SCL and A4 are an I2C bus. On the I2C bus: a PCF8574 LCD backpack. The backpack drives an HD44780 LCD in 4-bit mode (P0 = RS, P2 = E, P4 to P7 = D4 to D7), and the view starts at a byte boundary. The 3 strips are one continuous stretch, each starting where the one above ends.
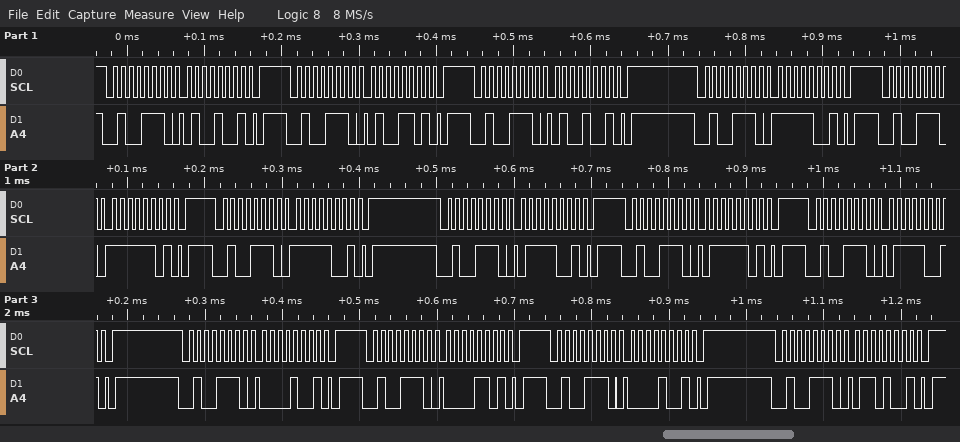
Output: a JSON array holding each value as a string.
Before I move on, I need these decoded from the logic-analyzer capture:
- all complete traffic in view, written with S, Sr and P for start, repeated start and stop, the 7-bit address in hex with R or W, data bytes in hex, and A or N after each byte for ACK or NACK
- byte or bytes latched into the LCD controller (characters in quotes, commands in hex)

["S 27W A 49 A P S 27W A 4D A P S 27W A 49 A P S 27W A F9 A P S 27W A FD A P S 27W A F9 A P S 27W A 79 A P S 27W A 7D A P S 27W A 79 A P S 27W A 09 A P S 27W A 0D A P S 27W A 09 A P S 27W A 69 A P", "'O' 'p'"]
